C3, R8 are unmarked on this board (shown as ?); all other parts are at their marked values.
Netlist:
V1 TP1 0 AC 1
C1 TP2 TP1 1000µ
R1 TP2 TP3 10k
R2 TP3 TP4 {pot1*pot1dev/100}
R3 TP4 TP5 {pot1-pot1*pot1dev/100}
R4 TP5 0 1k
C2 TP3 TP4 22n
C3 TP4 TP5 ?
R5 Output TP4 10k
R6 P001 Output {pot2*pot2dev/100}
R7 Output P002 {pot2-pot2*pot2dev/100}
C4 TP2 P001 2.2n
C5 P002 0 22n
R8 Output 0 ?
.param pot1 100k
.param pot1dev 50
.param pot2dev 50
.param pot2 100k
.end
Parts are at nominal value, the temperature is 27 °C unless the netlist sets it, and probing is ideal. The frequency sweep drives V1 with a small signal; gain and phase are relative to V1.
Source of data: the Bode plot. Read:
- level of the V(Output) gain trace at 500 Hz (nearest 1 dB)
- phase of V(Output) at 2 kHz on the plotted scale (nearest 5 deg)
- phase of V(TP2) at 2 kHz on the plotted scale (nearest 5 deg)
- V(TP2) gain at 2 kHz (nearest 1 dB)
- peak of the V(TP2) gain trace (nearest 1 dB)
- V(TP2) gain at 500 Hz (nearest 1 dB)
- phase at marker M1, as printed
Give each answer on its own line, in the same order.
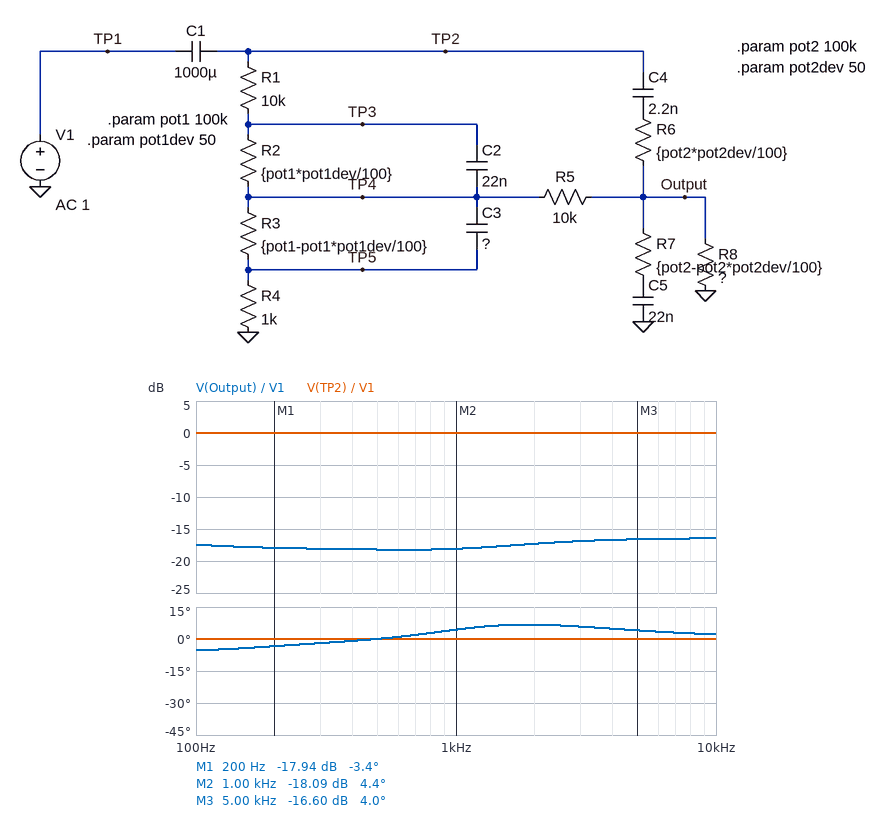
-18 dB
5 deg
0 deg
0 dB
0 dB
0 dB
-3.4 deg
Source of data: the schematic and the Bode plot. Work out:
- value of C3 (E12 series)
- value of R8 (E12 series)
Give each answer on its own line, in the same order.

68 nF
18 kΩ
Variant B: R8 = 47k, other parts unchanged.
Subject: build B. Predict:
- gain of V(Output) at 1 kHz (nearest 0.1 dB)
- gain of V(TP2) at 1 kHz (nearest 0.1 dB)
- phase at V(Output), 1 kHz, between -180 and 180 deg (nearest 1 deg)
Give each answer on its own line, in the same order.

-16.2 dB
0 dB
2 deg
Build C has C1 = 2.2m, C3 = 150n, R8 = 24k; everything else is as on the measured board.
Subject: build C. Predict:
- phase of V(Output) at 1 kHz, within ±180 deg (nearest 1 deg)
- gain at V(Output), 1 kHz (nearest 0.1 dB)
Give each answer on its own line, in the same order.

21 deg
-19.1 dB
